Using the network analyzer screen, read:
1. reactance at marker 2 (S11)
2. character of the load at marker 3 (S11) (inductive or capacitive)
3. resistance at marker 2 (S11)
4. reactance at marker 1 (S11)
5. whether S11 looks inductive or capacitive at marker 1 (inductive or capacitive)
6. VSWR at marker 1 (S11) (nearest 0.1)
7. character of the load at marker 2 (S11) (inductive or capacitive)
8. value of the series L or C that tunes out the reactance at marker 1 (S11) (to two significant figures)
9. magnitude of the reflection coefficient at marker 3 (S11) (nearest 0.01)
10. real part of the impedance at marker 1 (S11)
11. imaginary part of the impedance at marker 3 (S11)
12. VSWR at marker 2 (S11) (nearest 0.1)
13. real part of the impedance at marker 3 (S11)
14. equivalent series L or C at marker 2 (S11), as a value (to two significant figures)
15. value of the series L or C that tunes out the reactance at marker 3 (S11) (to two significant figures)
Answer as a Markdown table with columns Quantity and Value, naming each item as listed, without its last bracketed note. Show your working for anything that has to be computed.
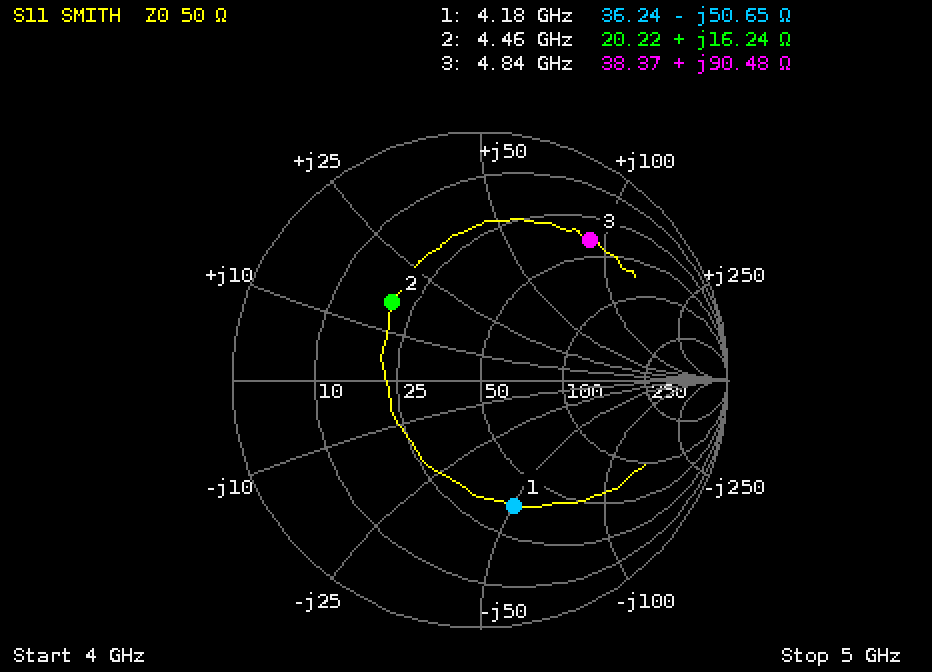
| Quantity | Value |
|---|---|
| reactance at marker 2 | +16.24 Ω |
| character of the load at marker 3 (S11) | inductive |
| resistance at marker 2 | 20.22 Ω |
| reactance at marker 1 | -50.65 Ω |
| whether S11 looks inductive or capacitive at marker 1 | capacitive |
| VSWR at marker 1 (S11) | 3.2 |
| character of the load at marker 2 (S11) | inductive |
| value of the series L or C that tunes out the reactance at marker 1 (S11) | L = 50.65 Ω/(2π × 4.18 GHz) ≈ 1.9 nH |
| magnitude of the reflection coefficient at marker 3 (S11) | 0.72 |
| real part of the impedance at marker 1 | 36.24 Ω |
| imaginary part of the impedance at marker 3 | +90.48 Ω |
| VSWR at marker 2 (S11) | 2.8 |
| real part of the impedance at marker 3 | 38.37 Ω |
| equivalent series L or C at marker 2 (S11), as a value | L = 16.24 Ω/(2π × 4.46 GHz) ≈ 580 pH |
| value of the series L or C that tunes out the reactance at marker 3 (S11) | C = 1/(2π × 4.84 GHz × 90.48 Ω) ≈ 363 fF, so 360 fF to two significant figures |
